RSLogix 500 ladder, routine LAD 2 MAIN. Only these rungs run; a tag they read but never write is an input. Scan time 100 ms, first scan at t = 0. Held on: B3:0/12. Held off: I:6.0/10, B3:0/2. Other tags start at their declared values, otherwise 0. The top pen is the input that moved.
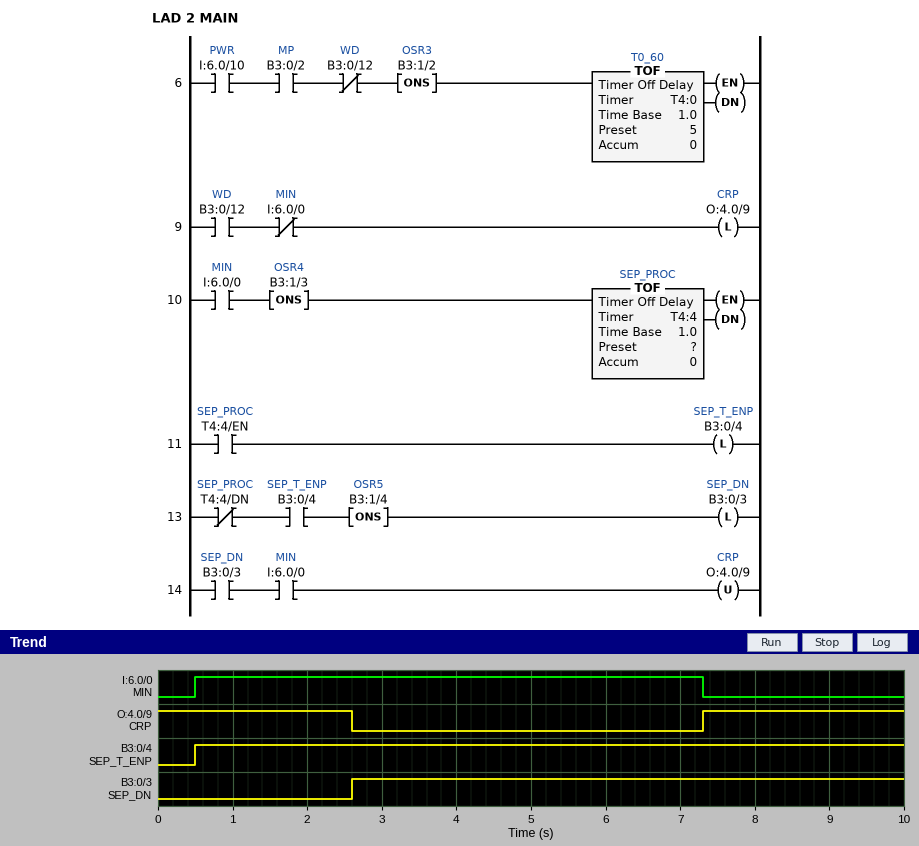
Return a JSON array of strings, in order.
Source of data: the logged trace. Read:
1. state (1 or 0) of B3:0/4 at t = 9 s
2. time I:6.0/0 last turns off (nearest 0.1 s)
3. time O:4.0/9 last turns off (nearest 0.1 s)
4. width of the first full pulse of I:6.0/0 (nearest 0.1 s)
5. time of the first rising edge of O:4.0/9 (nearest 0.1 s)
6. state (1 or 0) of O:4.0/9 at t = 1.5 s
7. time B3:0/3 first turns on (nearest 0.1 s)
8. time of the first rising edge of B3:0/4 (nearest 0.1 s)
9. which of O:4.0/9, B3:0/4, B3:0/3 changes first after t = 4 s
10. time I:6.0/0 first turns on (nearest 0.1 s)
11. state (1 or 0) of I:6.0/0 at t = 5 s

["1", "7.3 s", "2.6 s", "6.8 s", "7.3 s", "1", "2.6 s", "0.5 s", "O:4.0/9", "0.5 s", "1"]
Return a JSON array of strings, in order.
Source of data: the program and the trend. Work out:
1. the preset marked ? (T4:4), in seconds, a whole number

["2 s"]
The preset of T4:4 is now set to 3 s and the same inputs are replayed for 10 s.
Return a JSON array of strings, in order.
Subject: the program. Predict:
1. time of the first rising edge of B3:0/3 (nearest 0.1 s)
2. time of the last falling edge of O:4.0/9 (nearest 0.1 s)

["3.6 s", "3.6 s"]
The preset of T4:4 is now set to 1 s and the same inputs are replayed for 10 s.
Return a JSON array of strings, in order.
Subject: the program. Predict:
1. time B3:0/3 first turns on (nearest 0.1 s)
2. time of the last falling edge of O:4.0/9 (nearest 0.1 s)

["1.6 s", "1.6 s"]
